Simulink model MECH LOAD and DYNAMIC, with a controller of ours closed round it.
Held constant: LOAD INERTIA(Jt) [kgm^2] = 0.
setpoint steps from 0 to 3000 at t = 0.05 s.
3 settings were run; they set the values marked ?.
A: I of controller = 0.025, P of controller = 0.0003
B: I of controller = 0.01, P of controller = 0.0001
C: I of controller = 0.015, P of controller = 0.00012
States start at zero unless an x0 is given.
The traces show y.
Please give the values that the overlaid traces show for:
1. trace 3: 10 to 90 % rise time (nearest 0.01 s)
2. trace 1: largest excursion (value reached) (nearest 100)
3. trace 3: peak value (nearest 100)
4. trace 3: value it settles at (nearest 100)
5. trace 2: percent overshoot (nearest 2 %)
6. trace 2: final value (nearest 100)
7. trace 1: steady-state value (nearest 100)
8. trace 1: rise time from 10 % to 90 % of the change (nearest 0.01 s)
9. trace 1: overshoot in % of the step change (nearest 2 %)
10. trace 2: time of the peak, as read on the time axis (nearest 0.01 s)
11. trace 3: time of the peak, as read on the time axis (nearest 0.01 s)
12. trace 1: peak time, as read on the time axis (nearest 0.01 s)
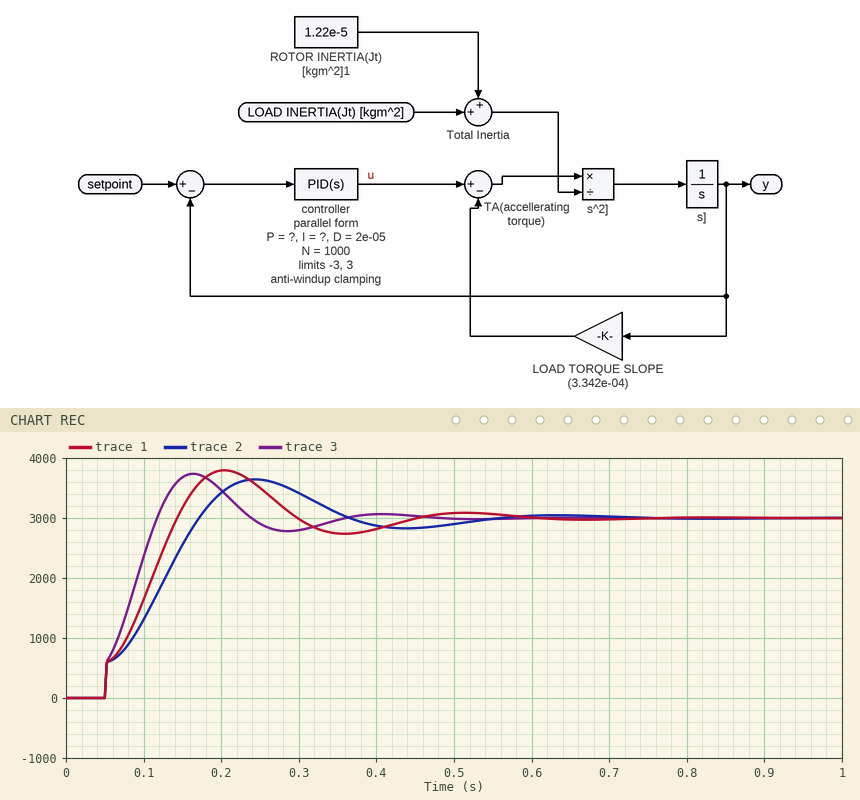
0.06 s
3800
3700
3000
22 %
3000
3000
0.08 s
26 %
0.24 s
0.16 s
0.20 s
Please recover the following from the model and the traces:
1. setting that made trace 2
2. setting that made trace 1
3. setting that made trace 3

B
C
A
